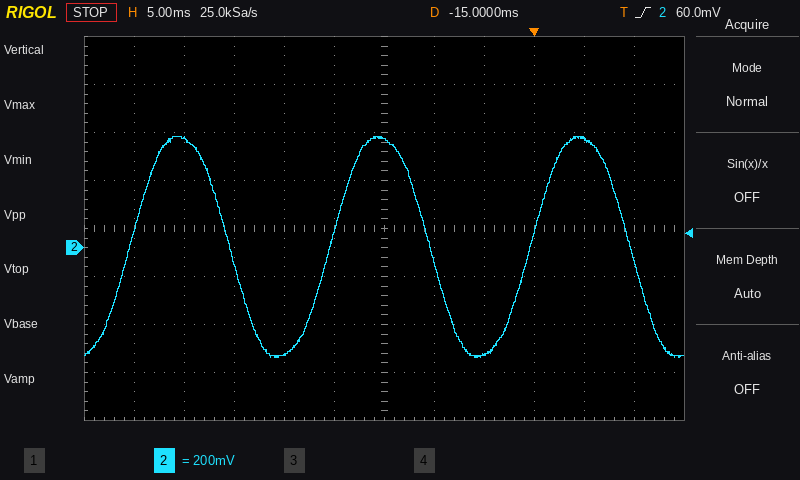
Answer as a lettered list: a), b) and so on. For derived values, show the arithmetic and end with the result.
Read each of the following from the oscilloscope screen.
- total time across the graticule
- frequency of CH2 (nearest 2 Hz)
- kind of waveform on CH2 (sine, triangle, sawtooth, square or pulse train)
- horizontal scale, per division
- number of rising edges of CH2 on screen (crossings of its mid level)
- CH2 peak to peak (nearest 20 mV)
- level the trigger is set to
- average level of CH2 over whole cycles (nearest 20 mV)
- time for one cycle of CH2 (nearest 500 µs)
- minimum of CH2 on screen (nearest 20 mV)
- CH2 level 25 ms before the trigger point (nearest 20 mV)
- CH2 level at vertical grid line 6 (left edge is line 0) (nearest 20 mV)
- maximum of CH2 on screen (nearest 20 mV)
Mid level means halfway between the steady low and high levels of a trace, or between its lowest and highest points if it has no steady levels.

a) 60 ms
b) 1 / 20.0 ms ≈ 50 Hz
c) sine
d) 5 ms
e) 3
f) 460 mV − (-460 mV) = 920 mV
g) 60.0 mV
h) (460 mV + (-460 mV)) / 2 ≈ 0 mV
i) 20.0 ms
j) -460 mV
k) -440 mV
l) 460 mV
m) 460 mV
